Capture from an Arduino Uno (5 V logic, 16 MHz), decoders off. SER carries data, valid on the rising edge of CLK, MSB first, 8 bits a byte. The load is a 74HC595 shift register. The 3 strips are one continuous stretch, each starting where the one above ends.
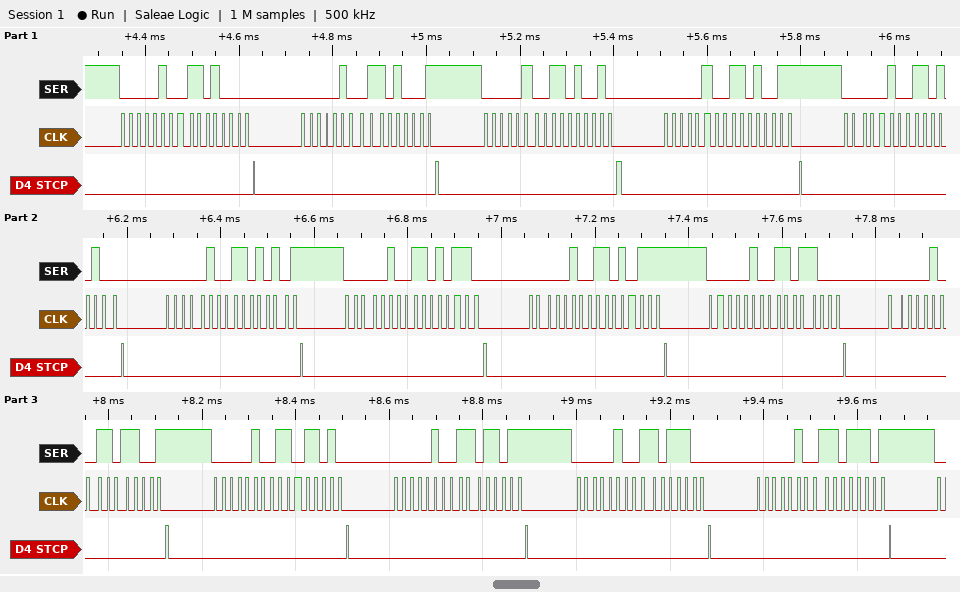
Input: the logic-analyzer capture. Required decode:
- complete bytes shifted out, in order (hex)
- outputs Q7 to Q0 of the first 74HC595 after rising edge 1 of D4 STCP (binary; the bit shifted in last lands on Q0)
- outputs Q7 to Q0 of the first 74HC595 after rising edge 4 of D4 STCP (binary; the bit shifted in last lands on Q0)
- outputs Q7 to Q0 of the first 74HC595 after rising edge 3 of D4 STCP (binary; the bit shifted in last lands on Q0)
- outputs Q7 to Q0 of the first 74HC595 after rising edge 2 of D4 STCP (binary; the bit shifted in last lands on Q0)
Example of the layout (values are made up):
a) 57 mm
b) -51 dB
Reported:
a) 0x04 0xD0 0x04 0xD1 0x04 0xD2 0x04 0xD3 0x04 0xD4 0x04 0xD5 0x04 0xD6 0x04 0xD7 0x04 0xD8 0x04 0xD9 0x04 0xDA 0x04 0xDB 0x04 0xDC 0x04 0xDD
b) 11010000
c) 11010011
d) 11010010
e) 11010001
